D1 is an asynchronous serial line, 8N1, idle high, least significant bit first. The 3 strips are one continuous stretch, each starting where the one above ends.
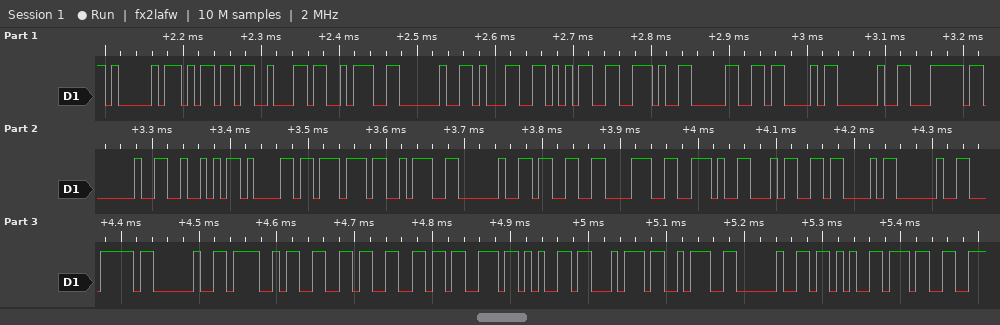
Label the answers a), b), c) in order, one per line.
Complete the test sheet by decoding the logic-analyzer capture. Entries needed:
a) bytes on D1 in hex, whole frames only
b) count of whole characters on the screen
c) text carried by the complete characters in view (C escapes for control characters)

a) 41 6D 62 3A 20 31 35 2E 30 43 20 7C 20 52 61 77 3A 20 33 38 2E 34 43 20 7C 20 4F 66 66 73 65 74 3A 20 2B 37
b) 36
c) "Amb: 15.0C | Raw: 38.4C | Offset: +7"
